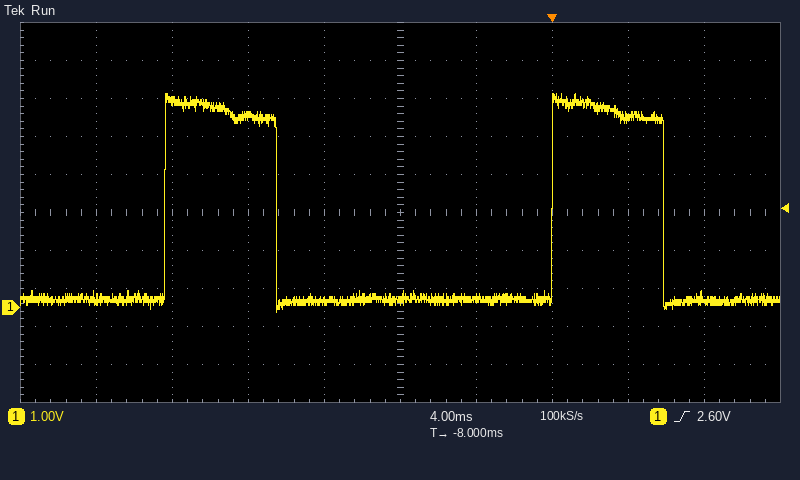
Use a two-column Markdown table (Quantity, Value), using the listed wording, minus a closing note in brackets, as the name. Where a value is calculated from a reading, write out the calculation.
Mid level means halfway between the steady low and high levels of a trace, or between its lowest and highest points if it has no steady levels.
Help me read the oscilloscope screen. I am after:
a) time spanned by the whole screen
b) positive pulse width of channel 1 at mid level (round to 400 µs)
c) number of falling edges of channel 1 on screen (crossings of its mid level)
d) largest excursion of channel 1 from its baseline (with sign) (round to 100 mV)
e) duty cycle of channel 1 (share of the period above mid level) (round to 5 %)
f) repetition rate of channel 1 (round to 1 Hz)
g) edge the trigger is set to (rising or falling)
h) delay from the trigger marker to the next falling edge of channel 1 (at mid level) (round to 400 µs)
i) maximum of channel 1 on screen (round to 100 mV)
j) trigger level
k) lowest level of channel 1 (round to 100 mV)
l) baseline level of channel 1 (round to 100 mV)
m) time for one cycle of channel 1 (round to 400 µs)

| Quantity | Value |
|---|---|
| time spanned by the whole screen | 40 ms |
| positive pulse width of channel 1 at mid level | 6.0 ms |
| number of falling edges of channel 1 on screen | 2 |
| largest excursion of channel 1 from its baseline (with sign) | 5.6 V − (200 mV) = +5.4 V |
| duty cycle of channel 1 (share of the period above mid level) | 6.0 ms / 20.4 ms ≈ 29.4 %, so 30 % to the nearest 5 % |
| repetition rate of channel 1 | 1 / 20.4 ms ≈ 49 Hz |
| edge the trigger is set to | rising |
| delay from the trigger marker to the next falling edge of channel 1 (at mid level) | 6.0 ms |
| maximum of channel 1 on screen | 5.6 V |
| trigger level | 2.60 V |
| lowest level of channel 1 | -100 mV |
| baseline level of channel 1 | 200 mV |
| time for one cycle of channel 1 | 20.4 ms |
